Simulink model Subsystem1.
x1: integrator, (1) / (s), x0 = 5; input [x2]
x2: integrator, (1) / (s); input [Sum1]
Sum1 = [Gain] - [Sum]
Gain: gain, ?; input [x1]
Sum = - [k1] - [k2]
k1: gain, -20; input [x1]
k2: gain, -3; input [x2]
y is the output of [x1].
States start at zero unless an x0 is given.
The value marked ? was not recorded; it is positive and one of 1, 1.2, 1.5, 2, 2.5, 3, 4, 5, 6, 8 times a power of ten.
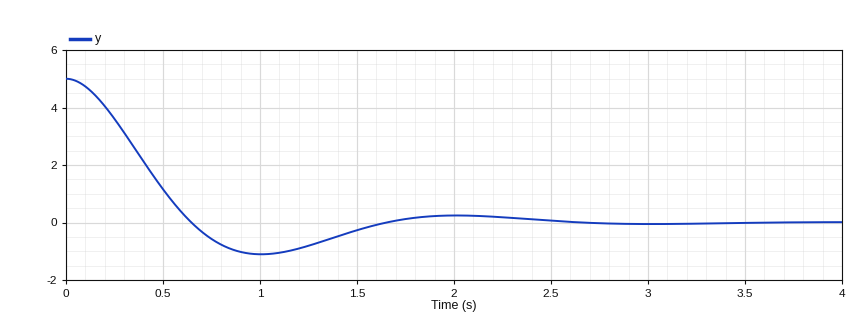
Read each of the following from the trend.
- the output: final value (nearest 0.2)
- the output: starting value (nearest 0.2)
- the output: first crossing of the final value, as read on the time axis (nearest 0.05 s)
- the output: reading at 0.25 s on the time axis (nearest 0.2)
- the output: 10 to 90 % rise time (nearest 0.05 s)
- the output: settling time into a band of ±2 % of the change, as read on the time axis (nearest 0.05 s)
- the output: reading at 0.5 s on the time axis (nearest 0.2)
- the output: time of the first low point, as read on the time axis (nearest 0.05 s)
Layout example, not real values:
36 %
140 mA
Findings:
0.0
5.0
0.65 s
3.6
0.45 s
2.40 s
1.2
1.00 s
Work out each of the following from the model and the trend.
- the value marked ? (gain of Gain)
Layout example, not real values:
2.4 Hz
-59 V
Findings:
8
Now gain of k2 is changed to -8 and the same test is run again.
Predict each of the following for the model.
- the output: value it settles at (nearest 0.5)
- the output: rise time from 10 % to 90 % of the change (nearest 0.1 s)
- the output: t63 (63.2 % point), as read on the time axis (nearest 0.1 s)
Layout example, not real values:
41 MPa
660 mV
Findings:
0.0
1.2 s
0.7 s
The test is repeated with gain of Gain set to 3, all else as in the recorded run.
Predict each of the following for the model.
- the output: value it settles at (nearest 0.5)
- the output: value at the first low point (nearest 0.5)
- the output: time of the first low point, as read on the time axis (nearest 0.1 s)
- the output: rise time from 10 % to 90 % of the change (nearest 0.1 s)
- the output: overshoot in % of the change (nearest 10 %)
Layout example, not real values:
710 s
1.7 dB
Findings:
0.0
-1.5
0.8 s
0.3 s
30 %
